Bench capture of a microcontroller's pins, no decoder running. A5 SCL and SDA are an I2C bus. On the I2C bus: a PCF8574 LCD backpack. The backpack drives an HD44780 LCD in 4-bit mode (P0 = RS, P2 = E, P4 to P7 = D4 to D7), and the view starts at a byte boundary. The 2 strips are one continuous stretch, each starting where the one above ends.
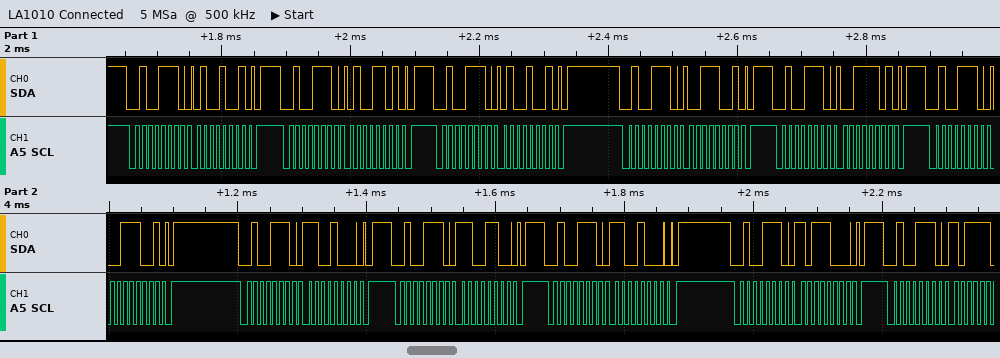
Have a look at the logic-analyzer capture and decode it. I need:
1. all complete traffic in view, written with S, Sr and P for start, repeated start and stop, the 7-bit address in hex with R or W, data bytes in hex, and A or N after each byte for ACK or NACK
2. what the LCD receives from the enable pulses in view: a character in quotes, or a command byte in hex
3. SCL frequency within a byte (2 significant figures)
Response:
S 27W A 49 A P S 27W A 4D A P S 27W A 49 A P S 27W A 39 A P S 27W A 3D A P S 27W A 39 A P S 27W A C8 A P S 27W A CC A P S 27W A C8 A P S 27W A B8 A P S 27W A
'C'
100 kHz
